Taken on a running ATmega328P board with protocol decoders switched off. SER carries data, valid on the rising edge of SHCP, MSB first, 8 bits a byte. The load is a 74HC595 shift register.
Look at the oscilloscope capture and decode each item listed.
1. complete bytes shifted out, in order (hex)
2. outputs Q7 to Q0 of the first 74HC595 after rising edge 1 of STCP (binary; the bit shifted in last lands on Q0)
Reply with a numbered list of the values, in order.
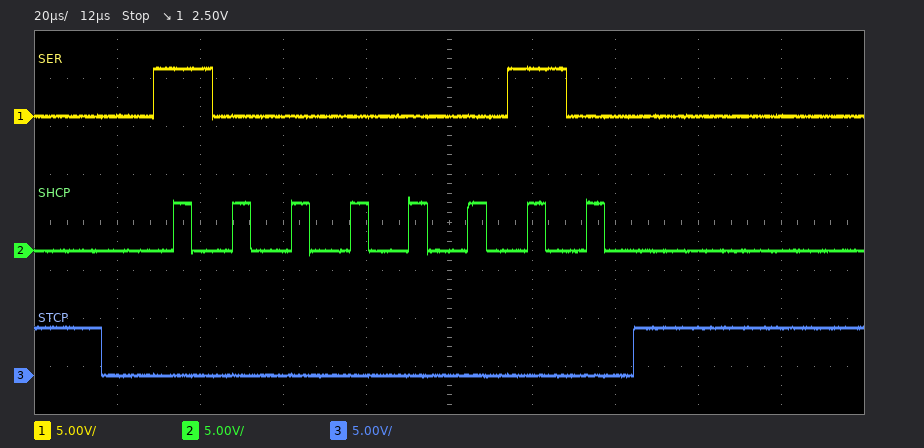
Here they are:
1. 0x82
2. 10000010
